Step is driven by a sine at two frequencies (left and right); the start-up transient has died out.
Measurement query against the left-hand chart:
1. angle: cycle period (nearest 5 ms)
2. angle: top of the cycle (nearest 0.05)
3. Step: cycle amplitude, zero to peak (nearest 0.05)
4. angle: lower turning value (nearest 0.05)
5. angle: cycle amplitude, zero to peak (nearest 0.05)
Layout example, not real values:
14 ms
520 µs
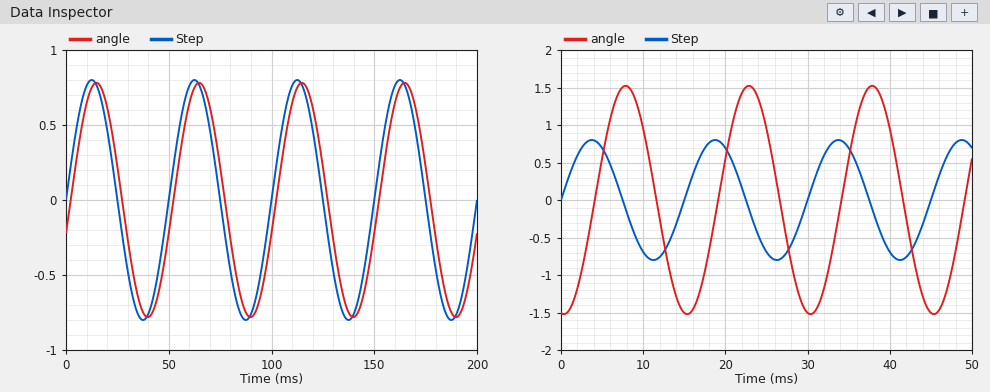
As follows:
50 ms
0.80
0.80
-0.80
0.80
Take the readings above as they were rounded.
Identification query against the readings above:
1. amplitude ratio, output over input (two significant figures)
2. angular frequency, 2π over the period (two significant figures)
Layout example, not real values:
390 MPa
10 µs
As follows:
1.0
0.13 rad/ms
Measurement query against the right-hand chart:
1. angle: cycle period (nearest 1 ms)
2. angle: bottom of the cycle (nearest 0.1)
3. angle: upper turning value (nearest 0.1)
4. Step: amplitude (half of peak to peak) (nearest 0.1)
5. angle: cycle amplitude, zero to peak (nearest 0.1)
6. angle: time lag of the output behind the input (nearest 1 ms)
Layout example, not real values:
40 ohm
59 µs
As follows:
15 ms
-1.5
1.5
0.8
1.5
4 ms
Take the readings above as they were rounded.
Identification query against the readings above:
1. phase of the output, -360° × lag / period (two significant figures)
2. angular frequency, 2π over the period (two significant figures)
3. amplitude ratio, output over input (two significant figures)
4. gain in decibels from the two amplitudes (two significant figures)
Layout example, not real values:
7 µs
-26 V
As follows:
-96°
0.42 rad/ms
1.9
5.5 dB
